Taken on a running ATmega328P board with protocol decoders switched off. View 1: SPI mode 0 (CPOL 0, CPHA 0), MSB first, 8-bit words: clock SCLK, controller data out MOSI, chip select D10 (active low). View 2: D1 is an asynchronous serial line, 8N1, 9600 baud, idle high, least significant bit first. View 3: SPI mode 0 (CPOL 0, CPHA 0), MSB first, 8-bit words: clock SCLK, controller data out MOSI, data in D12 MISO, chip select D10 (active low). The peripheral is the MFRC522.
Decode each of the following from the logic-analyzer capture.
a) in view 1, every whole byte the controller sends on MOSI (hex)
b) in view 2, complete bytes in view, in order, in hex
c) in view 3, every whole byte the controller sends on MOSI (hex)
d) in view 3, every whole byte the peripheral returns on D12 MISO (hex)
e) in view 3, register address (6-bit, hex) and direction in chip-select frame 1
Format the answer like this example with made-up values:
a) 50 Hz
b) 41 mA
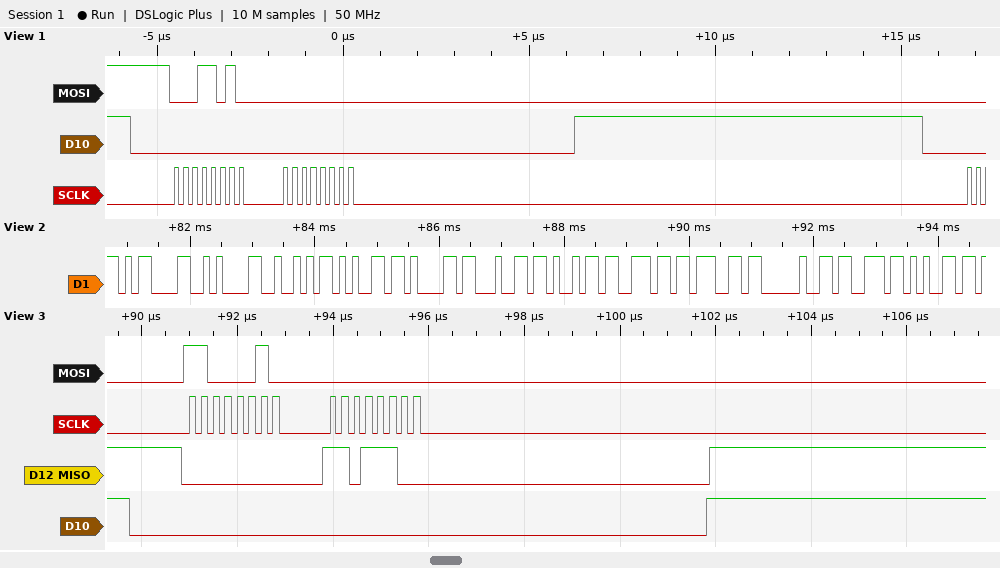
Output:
a) 1A 00
b) 0D 0A 52 65 61 64 69 6E 67 20 73 65
c) C2 00
d) 00 DC
e) 0x21 read
